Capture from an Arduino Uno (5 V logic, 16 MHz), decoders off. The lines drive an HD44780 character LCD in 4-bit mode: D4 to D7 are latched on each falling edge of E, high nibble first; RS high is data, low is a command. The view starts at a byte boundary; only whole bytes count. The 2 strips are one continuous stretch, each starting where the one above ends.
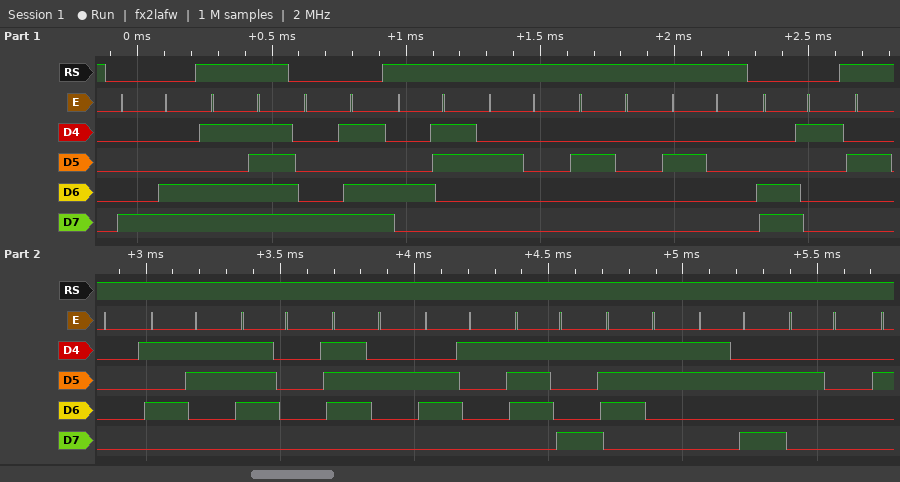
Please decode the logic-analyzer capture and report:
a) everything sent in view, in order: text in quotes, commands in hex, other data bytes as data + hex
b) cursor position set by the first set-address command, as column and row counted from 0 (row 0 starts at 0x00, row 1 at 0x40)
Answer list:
0x8C data DF 0x8D "C   " 0xC1 " Sprays: "
column 12, row 0
